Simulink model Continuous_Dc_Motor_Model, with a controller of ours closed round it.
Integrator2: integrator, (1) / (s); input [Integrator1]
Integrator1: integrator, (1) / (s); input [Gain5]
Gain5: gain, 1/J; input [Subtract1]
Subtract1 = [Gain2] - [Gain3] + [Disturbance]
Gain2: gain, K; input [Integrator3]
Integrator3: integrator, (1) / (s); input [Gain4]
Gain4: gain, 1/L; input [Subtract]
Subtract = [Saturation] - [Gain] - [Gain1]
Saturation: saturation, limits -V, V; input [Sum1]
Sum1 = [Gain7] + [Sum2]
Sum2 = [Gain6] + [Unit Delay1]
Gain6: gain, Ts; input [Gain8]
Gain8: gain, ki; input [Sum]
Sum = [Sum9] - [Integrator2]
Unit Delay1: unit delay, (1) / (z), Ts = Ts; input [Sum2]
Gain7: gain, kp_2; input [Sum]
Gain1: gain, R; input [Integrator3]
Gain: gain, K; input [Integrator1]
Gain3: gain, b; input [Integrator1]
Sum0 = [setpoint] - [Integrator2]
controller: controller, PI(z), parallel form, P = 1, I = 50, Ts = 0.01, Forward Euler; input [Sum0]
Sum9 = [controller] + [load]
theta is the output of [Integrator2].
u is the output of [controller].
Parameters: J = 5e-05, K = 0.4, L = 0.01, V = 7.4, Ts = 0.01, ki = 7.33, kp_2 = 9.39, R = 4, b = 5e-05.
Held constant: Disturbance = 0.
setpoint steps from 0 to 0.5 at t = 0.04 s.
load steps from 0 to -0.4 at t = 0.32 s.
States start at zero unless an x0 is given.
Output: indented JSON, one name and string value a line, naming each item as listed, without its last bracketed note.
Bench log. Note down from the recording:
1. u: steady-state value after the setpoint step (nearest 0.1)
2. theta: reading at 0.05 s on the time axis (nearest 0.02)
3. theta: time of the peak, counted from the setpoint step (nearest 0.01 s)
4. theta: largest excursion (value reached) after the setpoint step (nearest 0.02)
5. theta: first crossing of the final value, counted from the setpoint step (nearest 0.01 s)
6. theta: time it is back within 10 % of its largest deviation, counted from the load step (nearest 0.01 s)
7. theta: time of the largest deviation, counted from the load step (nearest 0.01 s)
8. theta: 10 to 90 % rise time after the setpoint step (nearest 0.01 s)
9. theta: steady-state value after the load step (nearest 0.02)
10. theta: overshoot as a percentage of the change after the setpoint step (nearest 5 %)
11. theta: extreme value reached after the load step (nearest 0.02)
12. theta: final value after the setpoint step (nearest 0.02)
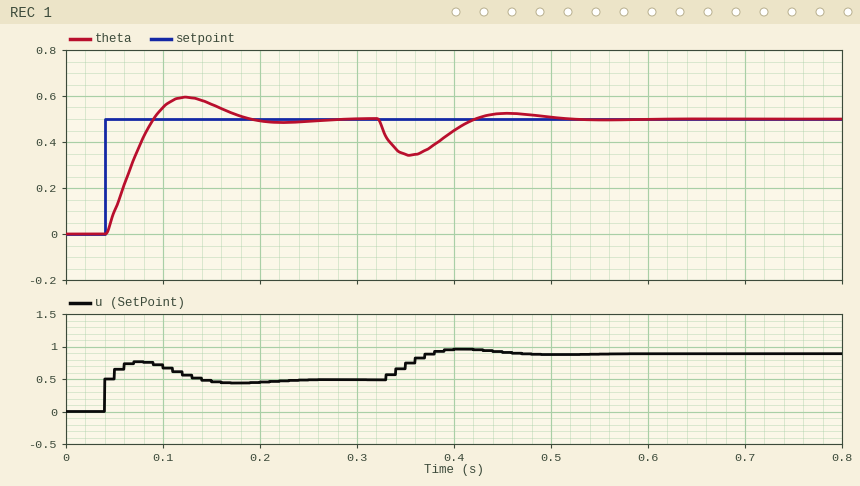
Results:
{
  "u: steady-state value after the setpoint step": "0.5",
  "theta: reading at 0.05 s on the time axis": "0.10",
  "theta: time of the peak, counted from the setpoint step": "0.08 s",
  "theta: largest excursion (value reached) after the setpoint step": "0.60",
  "theta: first crossing of the final value, counted from the setpoint step": "0.05 s",
  "theta: time it is back within 10 % of its largest deviation, counted from the load step": "0.16 s",
  "theta: time of the largest deviation, counted from the load step": "0.03 s",
  "theta: 10 to 90 % rise time after the setpoint step": "0.04 s",
  "theta: steady-state value after the load step": "0.50",
  "theta: overshoot as a percentage of the change after the setpoint step": "20 %",
  "theta: extreme value reached after the load step": "0.34",
  "theta: final value after the setpoint step": "0.50"
}
